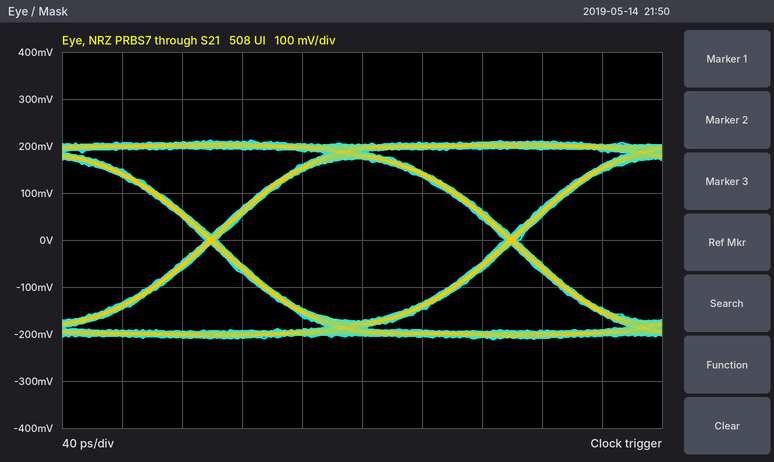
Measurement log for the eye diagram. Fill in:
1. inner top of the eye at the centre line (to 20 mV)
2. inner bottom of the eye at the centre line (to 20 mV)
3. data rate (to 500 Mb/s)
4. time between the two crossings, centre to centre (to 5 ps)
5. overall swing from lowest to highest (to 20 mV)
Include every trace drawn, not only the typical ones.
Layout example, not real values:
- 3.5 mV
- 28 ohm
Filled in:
- 180 mV
- -180 mV
- 5.0 Gb/s
- 200 ps
- 420 mV
